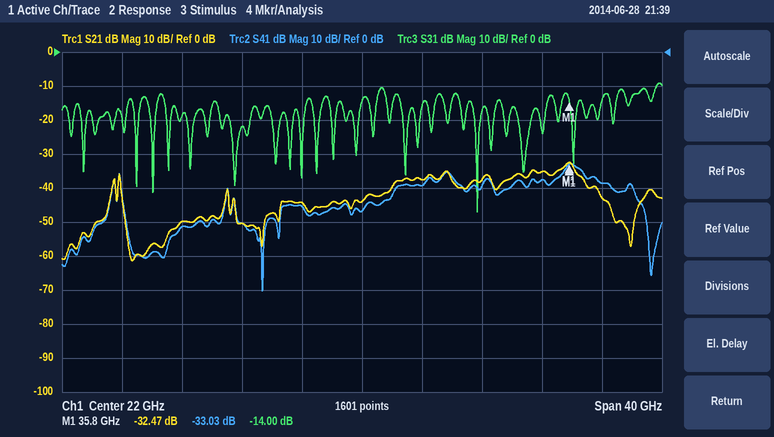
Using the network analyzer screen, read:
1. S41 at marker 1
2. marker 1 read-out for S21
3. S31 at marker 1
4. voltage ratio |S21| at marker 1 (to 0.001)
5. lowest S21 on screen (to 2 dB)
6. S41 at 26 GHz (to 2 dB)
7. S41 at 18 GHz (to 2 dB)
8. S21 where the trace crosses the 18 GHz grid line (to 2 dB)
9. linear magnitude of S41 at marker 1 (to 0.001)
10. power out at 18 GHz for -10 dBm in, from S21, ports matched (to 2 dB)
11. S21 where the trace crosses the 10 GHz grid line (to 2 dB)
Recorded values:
-33.03 dB
-32.47 dB
-14.00 dB
0.024
-62 dB
-40 dB
-46 dB
-44 dB
0.022
-54 dBm
-50 dB
